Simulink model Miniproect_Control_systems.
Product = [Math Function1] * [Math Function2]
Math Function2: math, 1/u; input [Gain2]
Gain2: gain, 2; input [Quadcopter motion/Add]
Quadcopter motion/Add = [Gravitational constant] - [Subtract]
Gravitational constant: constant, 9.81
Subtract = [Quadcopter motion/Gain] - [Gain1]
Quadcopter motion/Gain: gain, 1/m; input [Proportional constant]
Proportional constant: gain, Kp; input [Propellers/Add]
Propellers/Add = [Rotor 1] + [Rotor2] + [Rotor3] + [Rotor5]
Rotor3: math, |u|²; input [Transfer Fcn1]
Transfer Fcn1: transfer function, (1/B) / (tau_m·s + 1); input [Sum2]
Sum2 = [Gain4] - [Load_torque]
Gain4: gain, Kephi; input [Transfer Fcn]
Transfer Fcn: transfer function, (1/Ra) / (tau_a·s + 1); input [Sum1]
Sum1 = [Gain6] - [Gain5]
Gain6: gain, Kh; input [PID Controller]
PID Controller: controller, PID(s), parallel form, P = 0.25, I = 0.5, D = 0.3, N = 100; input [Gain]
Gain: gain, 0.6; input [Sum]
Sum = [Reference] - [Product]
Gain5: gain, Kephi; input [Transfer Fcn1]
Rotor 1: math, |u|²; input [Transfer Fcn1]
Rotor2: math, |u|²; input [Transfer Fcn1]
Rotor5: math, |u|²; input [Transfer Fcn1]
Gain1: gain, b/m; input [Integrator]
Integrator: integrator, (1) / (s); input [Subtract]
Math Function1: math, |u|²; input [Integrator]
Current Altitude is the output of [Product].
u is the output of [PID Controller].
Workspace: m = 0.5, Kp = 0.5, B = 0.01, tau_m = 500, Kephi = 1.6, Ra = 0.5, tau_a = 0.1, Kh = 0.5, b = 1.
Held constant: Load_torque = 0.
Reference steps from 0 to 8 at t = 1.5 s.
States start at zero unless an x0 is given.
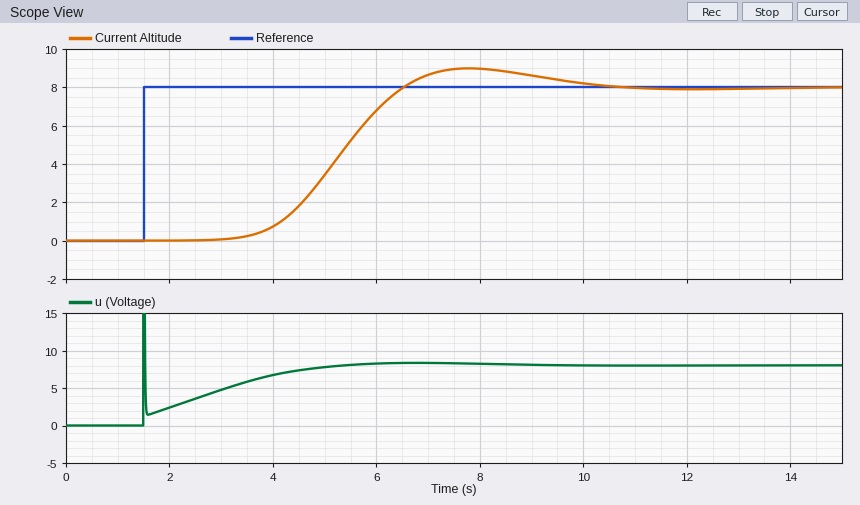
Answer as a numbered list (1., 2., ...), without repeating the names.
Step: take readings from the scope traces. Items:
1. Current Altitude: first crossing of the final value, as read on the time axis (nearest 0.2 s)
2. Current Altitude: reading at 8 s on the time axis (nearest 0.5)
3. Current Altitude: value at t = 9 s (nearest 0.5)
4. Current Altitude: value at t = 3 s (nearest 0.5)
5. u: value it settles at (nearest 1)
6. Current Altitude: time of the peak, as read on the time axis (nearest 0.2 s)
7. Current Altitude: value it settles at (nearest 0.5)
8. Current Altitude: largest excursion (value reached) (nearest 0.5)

1. 6.6 s
2. 9.0
3. 8.5
4. 0.0
5. 8
6. 7.8 s
7. 8.0
8. 9.0
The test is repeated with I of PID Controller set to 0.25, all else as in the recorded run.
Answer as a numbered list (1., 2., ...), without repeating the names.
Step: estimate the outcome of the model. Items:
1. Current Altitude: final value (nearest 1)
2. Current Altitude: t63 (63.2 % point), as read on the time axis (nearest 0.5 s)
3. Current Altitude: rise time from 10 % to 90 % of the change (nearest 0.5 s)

1. 8
2. 9.0 s
3. 5.5 s
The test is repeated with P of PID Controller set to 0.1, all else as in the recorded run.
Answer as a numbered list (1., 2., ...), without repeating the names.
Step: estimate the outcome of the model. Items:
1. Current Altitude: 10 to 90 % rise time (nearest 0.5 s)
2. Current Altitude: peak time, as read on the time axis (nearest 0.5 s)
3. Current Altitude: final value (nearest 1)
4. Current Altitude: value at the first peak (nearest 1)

1. 2.0 s
2. 7.5 s
3. 8
4. 10
